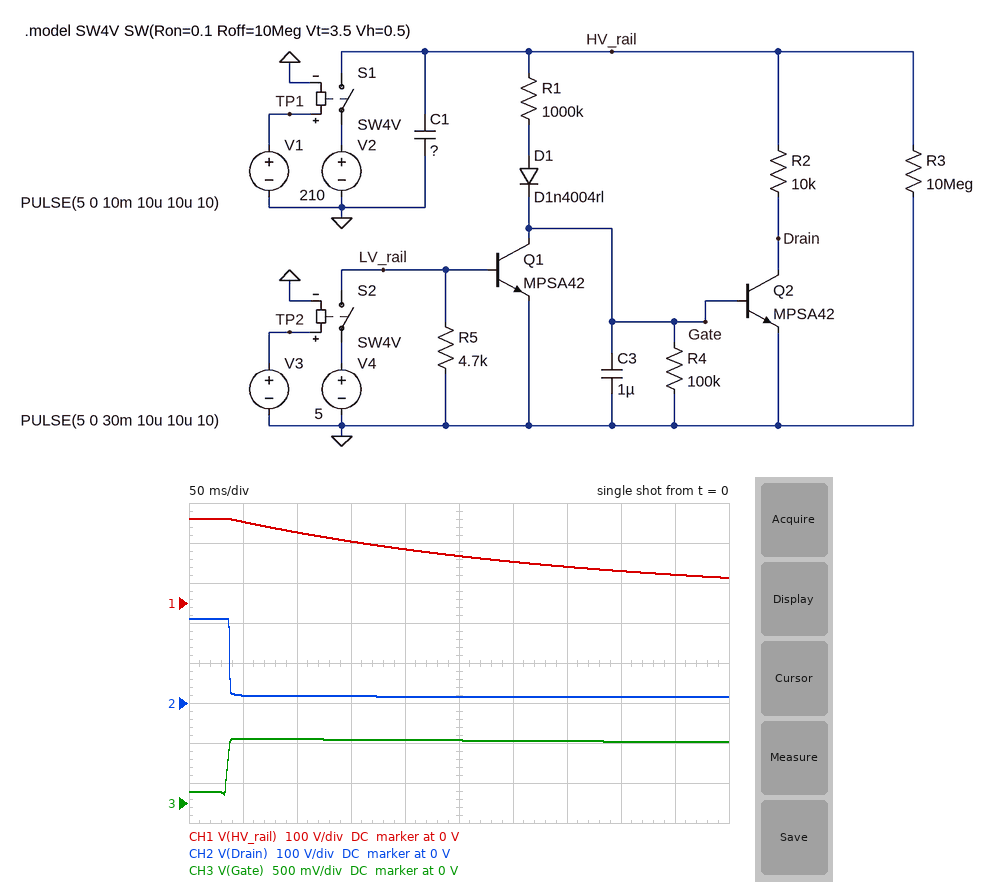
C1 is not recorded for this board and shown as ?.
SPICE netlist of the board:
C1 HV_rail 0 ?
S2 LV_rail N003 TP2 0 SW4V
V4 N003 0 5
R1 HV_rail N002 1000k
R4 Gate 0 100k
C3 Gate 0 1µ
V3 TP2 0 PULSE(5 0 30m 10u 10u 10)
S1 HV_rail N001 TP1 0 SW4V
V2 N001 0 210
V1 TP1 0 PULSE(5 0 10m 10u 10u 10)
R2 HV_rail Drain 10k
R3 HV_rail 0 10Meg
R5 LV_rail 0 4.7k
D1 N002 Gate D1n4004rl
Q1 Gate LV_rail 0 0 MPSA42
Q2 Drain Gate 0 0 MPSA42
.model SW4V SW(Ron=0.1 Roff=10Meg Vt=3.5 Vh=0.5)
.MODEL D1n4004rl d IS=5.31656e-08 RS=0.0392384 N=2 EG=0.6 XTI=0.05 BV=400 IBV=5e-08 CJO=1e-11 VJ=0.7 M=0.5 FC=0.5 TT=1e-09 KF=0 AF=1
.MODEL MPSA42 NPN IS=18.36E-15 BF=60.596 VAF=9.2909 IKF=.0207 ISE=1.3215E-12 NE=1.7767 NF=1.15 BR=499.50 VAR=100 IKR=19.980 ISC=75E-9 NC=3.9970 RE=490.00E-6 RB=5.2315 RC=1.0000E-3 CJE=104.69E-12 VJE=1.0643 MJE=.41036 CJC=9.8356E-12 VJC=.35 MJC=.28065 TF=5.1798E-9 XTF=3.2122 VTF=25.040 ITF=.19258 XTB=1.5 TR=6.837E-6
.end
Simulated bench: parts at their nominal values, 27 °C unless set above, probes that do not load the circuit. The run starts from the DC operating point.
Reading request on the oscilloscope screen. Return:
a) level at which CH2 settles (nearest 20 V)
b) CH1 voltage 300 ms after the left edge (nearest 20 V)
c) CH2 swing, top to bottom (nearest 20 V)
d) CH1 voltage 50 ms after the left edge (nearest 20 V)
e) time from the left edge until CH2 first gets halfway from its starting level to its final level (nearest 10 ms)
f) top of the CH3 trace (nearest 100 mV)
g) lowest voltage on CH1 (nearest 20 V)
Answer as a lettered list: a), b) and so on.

a) 20 V
b) 100 V
c) 200 V
d) 200 V
e) 40 ms
f) 800 mV
g) 60 V
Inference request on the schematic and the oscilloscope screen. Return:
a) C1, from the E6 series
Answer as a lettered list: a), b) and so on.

a) 33 µF
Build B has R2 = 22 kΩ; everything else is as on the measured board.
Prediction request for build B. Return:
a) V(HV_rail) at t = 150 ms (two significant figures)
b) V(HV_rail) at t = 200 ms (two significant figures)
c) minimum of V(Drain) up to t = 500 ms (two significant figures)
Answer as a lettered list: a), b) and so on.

a) 180 V
b) 170 V
c) 3.8 V
